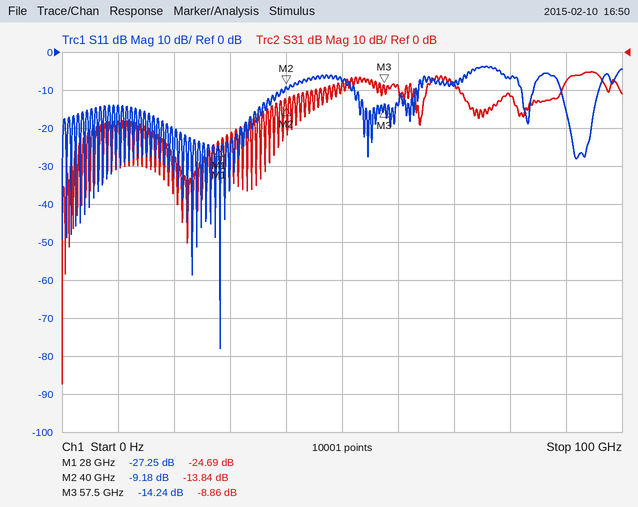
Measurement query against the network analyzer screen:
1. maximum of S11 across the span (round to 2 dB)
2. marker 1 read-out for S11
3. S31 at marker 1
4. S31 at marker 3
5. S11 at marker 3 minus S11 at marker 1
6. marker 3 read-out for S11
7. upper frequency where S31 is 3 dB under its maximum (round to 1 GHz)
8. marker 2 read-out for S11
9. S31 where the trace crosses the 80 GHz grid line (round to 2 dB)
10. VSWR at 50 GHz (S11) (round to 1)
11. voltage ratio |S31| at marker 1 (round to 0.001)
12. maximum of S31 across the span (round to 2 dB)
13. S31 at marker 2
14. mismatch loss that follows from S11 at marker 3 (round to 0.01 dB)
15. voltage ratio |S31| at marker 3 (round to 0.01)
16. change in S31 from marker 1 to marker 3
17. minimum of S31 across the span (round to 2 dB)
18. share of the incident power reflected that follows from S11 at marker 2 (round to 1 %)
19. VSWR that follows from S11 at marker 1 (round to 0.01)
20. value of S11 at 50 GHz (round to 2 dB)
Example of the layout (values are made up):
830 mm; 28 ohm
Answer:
-4 dB; -27.25 dB; -24.69 dB; -8.86 dB; 13.01 dB; -14.24 dB; 97 GHz; -9.18 dB; -12 dB; 2; 0.058; -6 dB; -13.84 dB; 0.17 dB; 0.36; 15.83 dB; -88 dB; 12 %; 1.09; -8 dB
